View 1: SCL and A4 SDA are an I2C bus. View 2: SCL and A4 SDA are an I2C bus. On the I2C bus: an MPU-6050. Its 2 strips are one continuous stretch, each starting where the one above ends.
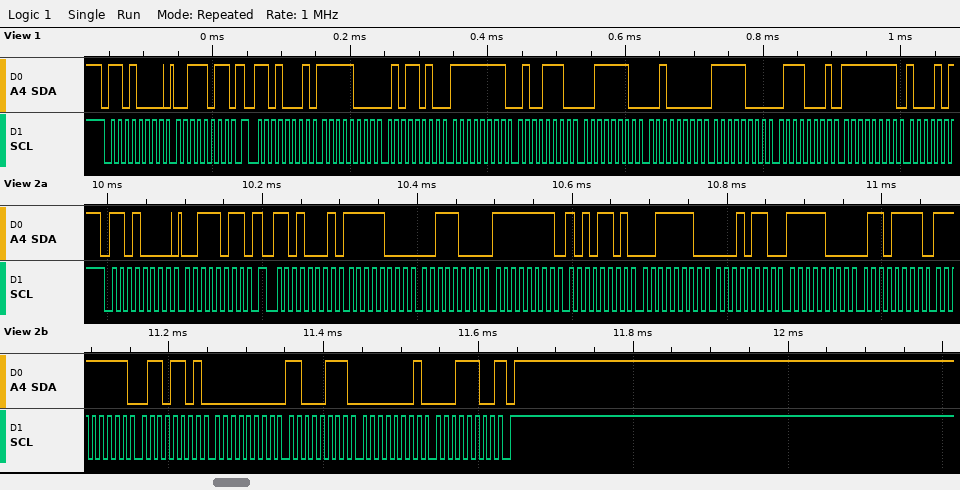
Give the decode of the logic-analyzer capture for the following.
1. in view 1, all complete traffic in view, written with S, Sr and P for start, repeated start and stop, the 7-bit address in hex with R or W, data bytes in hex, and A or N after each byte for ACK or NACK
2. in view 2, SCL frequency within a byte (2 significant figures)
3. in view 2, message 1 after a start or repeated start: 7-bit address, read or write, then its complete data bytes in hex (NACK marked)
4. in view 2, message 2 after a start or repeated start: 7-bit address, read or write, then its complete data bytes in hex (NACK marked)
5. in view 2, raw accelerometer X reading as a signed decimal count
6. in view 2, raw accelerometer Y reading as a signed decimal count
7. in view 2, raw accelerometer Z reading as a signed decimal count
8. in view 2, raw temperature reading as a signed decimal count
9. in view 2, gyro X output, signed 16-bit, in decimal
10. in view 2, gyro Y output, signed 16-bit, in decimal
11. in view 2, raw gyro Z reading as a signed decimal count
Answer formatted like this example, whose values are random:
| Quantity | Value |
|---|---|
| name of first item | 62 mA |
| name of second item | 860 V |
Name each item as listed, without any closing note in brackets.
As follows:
| Quantity | Value |
|---|---|
| in view 1, all complete traffic in view, written with S, Sr and P for start, repeated start and stop, the 7-bit address in hex with R or W, data bytes in hex, and A or N after each byte for ACK or NACK | S 68W A 3B A Sr 68R A F8 A 5A A FF A 4E A 3E A 20 A F8 A 71 A FF A |
| in view 2, SCL frequency within a byte | 100 kHz |
| in view 2, message 1 after a start or repeated start: 7-bit address, read or write, then its complete data bytes in hex | 0x68 write: 3B |
| in view 2, message 2 after a start or repeated start: 7-bit address, read or write, then its complete data bytes in hex | 0x68 read: F8 38 FF AD 3E 16 F8 6F FF 6D 00 C7 01 1C NACK |
| in view 2, raw accelerometer X reading as a signed decimal count | -1992 |
| in view 2, raw accelerometer Y reading as a signed decimal count | -83 |
| in view 2, raw accelerometer Z reading as a signed decimal count | 15894 |
| in view 2, raw temperature reading as a signed decimal count | -1937 |
| in view 2, gyro X output, signed 16-bit, in decimal | -147 |
| in view 2, gyro Y output, signed 16-bit, in decimal | 199 |
| in view 2, raw gyro Z reading as a signed decimal count | 284 |
